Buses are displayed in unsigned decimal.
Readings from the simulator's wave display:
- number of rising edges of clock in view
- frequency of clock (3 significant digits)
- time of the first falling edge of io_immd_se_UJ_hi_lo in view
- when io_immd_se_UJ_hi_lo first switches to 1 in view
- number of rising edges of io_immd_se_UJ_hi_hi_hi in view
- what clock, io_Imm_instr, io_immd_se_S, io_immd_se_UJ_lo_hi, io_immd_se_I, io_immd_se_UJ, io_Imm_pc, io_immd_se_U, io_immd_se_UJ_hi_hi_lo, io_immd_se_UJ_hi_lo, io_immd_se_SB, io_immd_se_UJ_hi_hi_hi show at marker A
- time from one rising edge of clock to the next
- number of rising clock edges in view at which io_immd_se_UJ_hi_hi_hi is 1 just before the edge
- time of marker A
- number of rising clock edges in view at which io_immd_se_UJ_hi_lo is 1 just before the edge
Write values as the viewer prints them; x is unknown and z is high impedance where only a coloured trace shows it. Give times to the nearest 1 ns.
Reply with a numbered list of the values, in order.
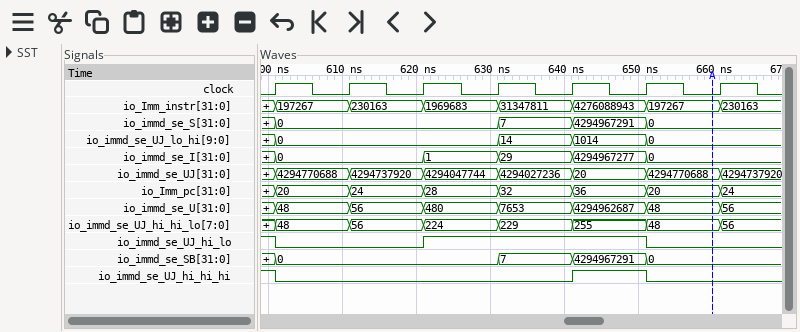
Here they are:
1. 7
2. 100 MHz
3. 601 ns
4. 621 ns
5. 1
6. clock=0, io_Imm_instr=197267, io_immd_se_S=0, io_immd_se_UJ_lo_hi=0, io_immd_se_I=0, io_immd_se_UJ=4294770688, io_Imm_pc=20, io_immd_se_U=48, io_immd_se_UJ_hi_hi_lo=48, io_immd_se_UJ_hi_lo=0, io_immd_se_SB=0, io_immd_se_UJ_hi_hi_hi=0
7. 10 ns
8. 2
9. 660 ns
10. 4
